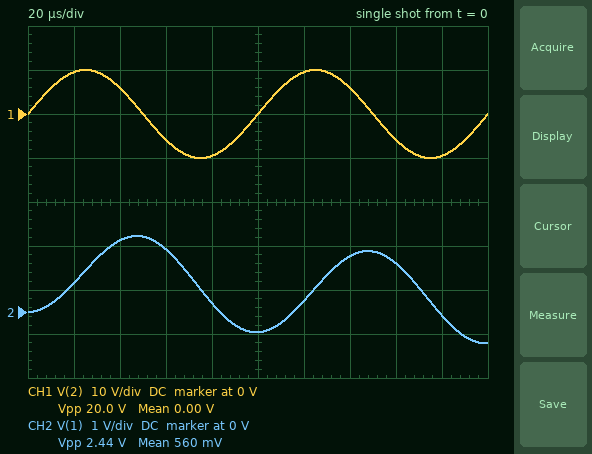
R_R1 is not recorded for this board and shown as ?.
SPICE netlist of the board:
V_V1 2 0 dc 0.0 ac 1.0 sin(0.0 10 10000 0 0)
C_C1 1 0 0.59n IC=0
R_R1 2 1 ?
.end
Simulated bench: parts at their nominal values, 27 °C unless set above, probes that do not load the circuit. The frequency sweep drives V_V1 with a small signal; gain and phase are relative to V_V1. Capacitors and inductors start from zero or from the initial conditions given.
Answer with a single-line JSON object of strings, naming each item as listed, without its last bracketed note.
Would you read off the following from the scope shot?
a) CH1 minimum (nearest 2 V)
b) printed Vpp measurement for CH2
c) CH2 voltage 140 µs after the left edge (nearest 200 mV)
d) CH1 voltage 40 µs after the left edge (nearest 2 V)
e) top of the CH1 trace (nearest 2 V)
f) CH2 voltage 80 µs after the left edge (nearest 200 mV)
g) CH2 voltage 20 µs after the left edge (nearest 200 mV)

{"CH1 minimum": "-10 V", "printed Vpp measurement for CH2": "2.44 V", "CH2 voltage 140 µs after the left edge": "1.2 V", "CH1 voltage 40 µs after the left edge": "6 V", "top of the CH1 trace": "10 V", "CH2 voltage 80 µs after the left edge": "200 mV", "CH2 voltage 20 µs after the left edge": "600 mV"}
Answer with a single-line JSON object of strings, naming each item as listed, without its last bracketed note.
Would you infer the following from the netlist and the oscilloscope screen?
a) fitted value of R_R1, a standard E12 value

{"fitted value of R_R1, a standard E12 value": "270 kΩ"}
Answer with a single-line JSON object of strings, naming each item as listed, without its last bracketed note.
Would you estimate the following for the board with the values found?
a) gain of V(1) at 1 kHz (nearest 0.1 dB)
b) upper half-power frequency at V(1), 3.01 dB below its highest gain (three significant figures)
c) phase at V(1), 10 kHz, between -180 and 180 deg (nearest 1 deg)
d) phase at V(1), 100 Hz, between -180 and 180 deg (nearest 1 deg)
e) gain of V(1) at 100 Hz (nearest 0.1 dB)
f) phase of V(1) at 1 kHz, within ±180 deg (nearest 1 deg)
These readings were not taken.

{"gain of V(1) at 1 kHz": "-3.0 dB", "upper half-power frequency at V(1), 3.01 dB below its highest gain": "999 Hz", "phase at V(1), 10 kHz, between -180 and 180 deg": "-84 deg", "phase at V(1), 100 Hz, between -180 and 180 deg": "-6 deg", "gain of V(1) at 100 Hz": "0 dB", "phase of V(1) at 1 kHz, within ±180 deg": "-45 deg"}
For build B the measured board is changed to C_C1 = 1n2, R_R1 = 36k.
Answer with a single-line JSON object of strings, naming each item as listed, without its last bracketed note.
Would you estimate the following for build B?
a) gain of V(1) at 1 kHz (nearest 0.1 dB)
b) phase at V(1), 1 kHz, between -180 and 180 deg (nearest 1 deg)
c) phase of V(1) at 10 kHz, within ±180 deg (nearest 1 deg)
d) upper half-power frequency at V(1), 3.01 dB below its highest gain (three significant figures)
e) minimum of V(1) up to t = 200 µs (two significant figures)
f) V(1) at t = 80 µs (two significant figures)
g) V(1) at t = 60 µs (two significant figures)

{"gain of V(1) at 1 kHz": "-0.3 dB", "phase at V(1), 1 kHz, between -180 and 180 deg": "-15 deg", "phase of V(1) at 10 kHz, within ±180 deg": "-70 deg", "upper half-power frequency at V(1), 3.01 dB below its highest gain": "3.68 kHz", "minimum of V(1) up to t = 200 µs": "-3.4 V", "V(1) at t = 80 µs": "-1.6 V", "V(1) at t = 60 µs": "2.7 V"}
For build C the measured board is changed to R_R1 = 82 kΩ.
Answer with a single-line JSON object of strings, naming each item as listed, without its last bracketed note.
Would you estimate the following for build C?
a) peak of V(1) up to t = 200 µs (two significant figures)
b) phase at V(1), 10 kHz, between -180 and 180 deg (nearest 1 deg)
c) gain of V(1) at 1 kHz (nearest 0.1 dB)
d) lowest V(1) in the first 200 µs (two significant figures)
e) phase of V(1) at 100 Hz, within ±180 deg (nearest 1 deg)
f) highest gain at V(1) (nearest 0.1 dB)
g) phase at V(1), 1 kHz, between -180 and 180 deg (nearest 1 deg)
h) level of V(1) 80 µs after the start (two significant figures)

{"peak of V(1) up to t = 200 µs": "4.3 V", "phase at V(1), 10 kHz, between -180 and 180 deg": "-72 deg", "gain of V(1) at 1 kHz": "-0.4 dB", "lowest V(1) in the first 200 µs": "-3.1 V", "phase of V(1) at 100 Hz, within ±180 deg": "-2 deg", "highest gain at V(1)": "0 dB", "phase at V(1), 1 kHz, between -180 and 180 deg": "-17 deg", "level of V(1) 80 µs after the start": "-1.3 V"}
